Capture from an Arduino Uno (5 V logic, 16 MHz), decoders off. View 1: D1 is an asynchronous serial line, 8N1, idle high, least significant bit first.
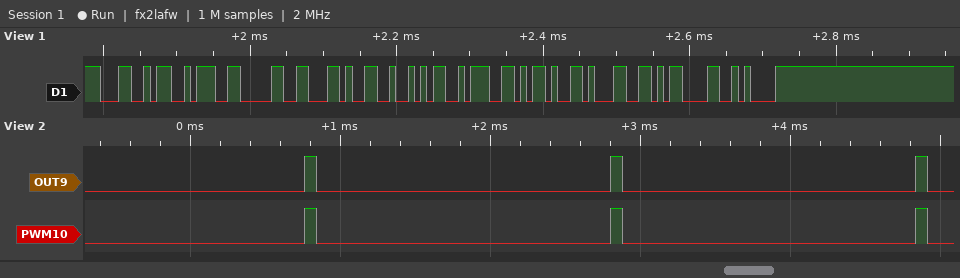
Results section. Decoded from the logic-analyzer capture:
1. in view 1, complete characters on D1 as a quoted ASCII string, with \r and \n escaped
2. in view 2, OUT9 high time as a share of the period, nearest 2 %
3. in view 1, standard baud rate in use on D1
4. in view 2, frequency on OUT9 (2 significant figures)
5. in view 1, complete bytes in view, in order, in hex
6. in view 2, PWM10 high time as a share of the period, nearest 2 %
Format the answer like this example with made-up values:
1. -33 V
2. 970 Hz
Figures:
1. "L:0,R:-1\r\n"
2. 4 %
3. 115200 baud
4. 490 Hz
5. 0x4C 0x3A 0x30 0x2C 0x52 0x3A 0x2D 0x31 0x0D 0x0A
6. 4 %
